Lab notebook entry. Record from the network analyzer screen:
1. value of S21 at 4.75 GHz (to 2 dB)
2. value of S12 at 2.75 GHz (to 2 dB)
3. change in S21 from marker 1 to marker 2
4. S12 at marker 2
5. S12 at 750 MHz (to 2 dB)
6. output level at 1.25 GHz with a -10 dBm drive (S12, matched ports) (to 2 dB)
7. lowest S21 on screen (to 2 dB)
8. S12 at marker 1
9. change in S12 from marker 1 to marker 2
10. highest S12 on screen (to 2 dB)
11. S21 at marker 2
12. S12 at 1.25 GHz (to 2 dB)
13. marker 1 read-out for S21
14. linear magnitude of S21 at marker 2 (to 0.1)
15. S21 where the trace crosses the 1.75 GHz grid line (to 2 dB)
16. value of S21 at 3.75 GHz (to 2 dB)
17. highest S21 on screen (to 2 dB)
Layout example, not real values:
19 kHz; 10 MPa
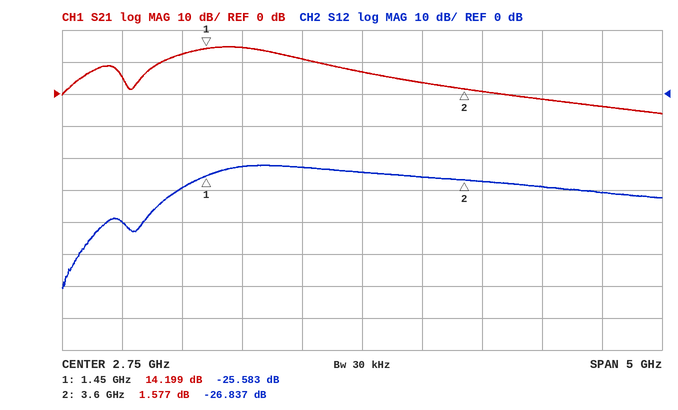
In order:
-4 dB; -24 dB; -12.622 dB; -26.837 dB; -40 dB; -40 dBm; -6 dB; -25.583 dB; -1.254 dB; -22 dB; 1.577 dB; -30 dB; 14.199 dB; 1.2; 14 dB; 0 dB; 14 dB
